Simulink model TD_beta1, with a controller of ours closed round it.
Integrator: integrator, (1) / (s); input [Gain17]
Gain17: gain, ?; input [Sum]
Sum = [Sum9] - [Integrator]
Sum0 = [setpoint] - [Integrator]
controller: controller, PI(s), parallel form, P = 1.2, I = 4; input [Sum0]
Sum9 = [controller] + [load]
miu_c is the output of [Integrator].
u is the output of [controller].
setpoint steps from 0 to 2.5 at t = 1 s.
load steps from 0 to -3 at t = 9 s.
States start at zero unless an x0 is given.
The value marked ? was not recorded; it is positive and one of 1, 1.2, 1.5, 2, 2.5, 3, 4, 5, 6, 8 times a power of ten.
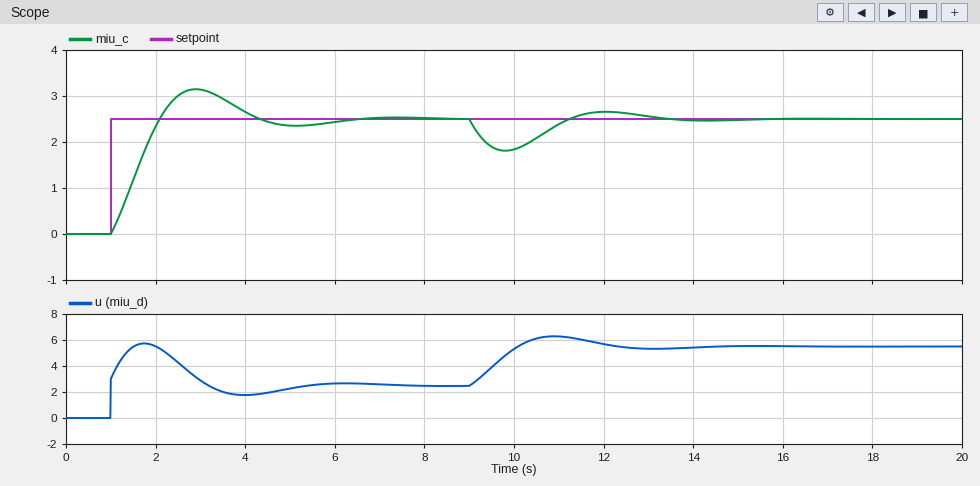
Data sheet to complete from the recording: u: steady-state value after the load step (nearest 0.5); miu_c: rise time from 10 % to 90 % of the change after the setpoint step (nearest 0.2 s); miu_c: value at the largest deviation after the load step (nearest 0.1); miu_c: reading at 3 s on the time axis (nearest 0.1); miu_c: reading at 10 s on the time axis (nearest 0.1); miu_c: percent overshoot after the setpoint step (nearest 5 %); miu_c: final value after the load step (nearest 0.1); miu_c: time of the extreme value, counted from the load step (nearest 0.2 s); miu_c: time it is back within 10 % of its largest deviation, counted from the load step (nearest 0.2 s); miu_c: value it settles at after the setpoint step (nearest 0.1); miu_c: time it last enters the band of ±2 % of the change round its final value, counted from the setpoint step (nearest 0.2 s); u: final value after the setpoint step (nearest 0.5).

5.5
0.8 s
1.8
3.1
1.8
25 %
2.5
0.8 s
4.0 s
2.5
5.2 s
2.5
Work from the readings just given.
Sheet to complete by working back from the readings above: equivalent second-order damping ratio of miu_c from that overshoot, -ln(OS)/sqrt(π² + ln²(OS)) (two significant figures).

0.40
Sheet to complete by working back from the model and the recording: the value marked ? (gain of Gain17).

0.6
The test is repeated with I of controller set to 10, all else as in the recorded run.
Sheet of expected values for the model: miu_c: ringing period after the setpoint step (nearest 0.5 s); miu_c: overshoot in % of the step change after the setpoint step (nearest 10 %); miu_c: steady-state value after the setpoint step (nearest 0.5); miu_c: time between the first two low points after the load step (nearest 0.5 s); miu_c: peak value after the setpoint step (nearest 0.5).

2.5 s
40 %
2.5
2.5 s
3.5
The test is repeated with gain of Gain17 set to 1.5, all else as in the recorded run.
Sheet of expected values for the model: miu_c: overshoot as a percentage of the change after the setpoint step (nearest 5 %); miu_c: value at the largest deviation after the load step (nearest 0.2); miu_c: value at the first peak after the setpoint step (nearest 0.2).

10 %
1.6
2.8
